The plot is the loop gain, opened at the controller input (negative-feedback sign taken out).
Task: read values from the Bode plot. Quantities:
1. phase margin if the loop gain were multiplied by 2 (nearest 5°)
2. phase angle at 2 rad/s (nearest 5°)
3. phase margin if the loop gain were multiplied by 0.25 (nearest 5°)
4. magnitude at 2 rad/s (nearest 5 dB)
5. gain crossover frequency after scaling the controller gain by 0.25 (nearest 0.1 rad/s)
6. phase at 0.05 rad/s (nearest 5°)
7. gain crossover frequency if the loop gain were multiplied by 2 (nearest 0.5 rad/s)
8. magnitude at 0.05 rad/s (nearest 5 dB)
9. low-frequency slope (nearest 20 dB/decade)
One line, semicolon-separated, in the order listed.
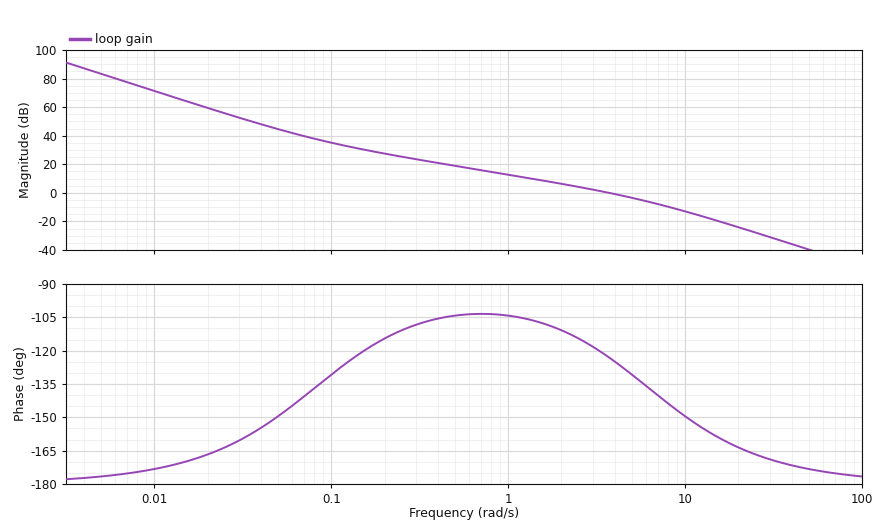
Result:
45°; -110°; 75°; 5 dB; 1.1 rad/s; -150°; 6.0 rad/s; 45 dB; -40 dB/decade
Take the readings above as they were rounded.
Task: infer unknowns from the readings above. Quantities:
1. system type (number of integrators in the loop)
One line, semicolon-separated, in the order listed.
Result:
2
